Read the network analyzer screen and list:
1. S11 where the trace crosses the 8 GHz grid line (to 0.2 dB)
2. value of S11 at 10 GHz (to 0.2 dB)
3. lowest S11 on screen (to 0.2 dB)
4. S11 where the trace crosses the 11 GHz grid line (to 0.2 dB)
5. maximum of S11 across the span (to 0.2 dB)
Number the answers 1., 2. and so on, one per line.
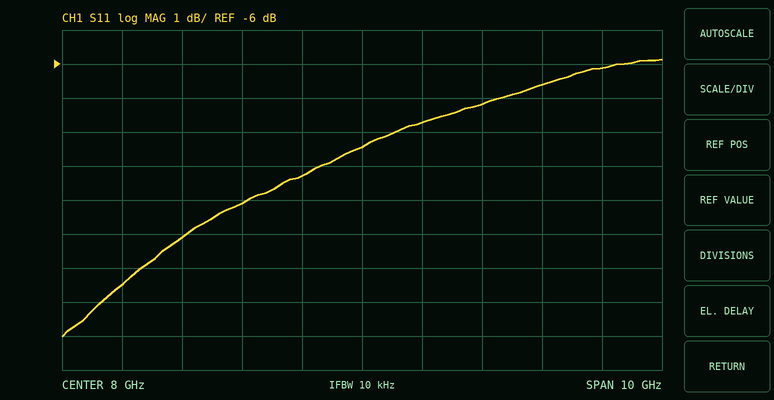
1. -8.4 dB
2. -7.2 dB
3. -14.0 dB
4. -6.6 dB
5. -5.8 dB
